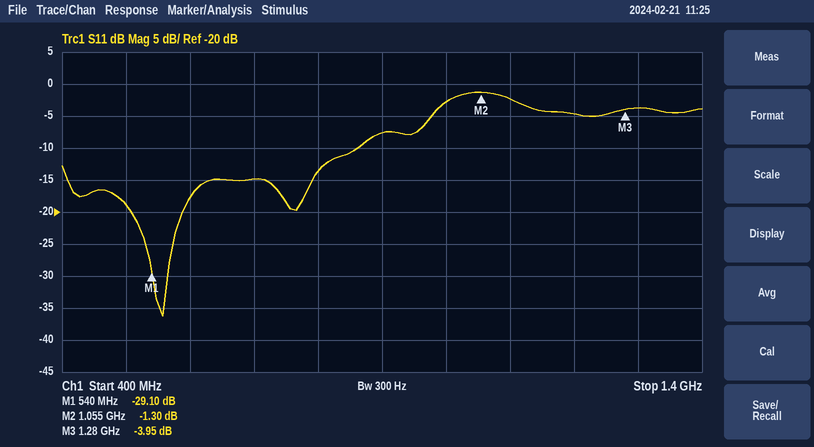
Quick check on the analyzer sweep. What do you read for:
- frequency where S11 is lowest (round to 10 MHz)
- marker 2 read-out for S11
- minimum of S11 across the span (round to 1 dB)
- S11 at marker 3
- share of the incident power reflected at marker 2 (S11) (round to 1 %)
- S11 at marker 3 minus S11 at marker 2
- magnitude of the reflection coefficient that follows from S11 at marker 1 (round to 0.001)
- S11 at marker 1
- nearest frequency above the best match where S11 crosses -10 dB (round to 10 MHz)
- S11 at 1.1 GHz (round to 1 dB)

560 MHz
-1.30 dB
-36 dB
-3.95 dB
74 %
-2.65 dB
0.035
-29.10 dB
860 MHz
-2 dB
